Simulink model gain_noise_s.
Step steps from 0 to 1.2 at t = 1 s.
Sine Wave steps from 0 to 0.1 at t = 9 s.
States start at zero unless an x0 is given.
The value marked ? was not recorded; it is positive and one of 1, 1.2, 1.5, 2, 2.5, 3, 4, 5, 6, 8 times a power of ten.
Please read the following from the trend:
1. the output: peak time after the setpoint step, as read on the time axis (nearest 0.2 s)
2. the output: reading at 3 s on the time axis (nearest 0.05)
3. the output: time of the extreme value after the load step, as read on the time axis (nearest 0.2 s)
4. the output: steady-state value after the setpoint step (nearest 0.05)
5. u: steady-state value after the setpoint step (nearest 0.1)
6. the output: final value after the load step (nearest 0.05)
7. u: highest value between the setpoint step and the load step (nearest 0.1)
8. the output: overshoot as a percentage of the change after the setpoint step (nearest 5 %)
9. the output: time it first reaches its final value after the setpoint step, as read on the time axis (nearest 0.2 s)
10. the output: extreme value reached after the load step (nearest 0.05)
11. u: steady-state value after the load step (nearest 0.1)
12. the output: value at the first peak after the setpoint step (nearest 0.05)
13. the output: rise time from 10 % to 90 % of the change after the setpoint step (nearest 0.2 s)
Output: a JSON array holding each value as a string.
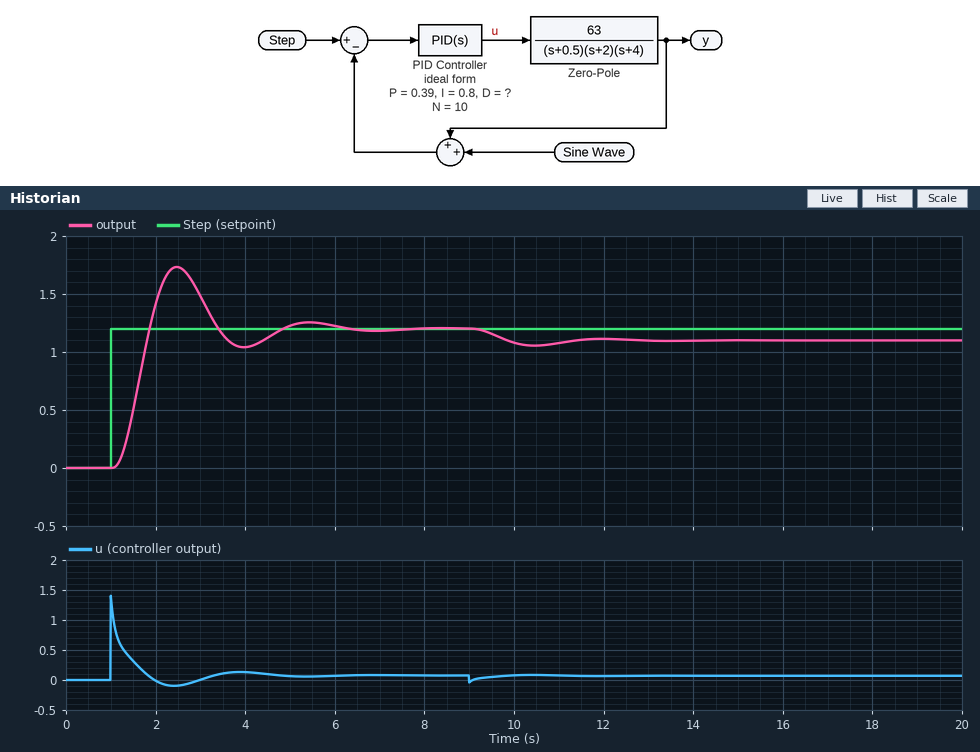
["2.4 s", "1.50", "10.4 s", "1.20", "0.1", "1.10", "1.4", "45 %", "1.8 s", "1.05", "0.1", "1.75", "0.6 s"]
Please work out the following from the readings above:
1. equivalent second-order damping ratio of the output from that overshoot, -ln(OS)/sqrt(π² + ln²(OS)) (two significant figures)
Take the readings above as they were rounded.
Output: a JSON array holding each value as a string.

["0.25"]
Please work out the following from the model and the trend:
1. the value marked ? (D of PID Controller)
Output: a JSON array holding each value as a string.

["0.2"]
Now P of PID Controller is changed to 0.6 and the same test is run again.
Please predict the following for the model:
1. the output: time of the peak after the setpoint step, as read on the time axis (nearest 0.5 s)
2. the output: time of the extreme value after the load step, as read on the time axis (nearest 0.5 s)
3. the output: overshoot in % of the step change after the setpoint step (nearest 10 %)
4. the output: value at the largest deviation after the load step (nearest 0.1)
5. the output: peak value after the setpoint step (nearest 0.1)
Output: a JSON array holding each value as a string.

["2.0 s", "10.0 s", "60 %", "1.0", "1.9"]
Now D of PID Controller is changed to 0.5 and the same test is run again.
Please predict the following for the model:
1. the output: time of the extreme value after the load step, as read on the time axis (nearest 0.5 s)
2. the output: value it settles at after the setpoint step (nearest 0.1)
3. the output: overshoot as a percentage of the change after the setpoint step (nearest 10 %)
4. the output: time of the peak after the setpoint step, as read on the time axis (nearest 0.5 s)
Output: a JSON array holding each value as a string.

["10.0 s", "1.2", "20 %", "2.0 s"]
